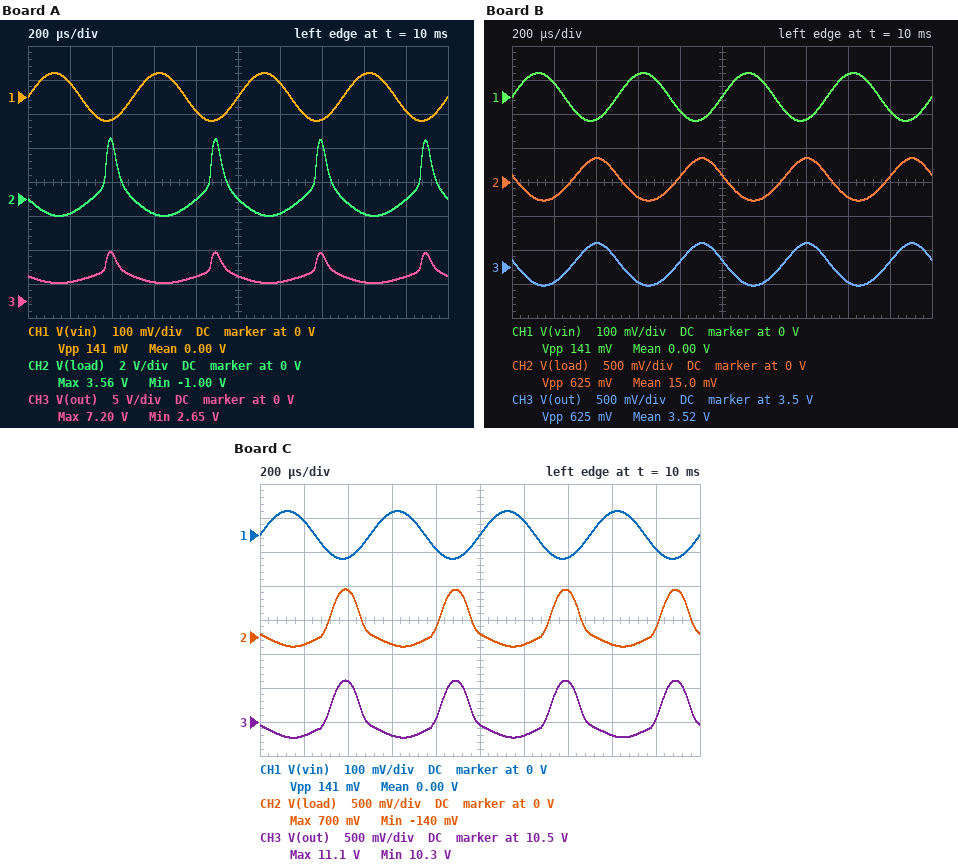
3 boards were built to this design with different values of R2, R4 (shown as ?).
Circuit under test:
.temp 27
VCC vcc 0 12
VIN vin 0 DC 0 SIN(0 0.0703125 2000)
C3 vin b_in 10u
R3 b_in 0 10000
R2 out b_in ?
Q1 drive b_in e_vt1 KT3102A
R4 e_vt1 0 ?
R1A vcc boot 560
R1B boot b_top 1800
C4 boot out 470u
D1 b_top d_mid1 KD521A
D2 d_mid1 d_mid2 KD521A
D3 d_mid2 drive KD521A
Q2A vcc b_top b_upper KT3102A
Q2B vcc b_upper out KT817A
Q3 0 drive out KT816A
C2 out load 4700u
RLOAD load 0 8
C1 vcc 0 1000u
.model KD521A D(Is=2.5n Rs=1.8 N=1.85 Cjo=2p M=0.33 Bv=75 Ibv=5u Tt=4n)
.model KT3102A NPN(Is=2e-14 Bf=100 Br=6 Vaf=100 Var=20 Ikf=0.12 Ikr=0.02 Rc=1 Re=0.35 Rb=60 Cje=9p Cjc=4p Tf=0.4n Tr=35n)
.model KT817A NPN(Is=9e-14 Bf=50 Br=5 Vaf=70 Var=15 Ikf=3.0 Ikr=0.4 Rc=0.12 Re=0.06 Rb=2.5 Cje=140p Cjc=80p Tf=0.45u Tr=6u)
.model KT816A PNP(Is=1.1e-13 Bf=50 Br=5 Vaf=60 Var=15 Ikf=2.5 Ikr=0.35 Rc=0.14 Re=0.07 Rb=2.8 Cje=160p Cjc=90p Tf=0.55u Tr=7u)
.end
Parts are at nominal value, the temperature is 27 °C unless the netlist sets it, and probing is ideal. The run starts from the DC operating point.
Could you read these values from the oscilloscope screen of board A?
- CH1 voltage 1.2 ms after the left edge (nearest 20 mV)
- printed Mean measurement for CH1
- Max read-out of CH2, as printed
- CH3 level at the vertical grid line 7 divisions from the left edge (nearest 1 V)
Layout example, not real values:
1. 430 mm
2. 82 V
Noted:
1. 40 mV
2. 0.00 V
3. 3.56 V
4. 7 V
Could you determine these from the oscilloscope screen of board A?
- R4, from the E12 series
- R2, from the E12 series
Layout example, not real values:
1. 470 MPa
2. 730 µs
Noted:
1. 33 Ω
2. 22 kΩ
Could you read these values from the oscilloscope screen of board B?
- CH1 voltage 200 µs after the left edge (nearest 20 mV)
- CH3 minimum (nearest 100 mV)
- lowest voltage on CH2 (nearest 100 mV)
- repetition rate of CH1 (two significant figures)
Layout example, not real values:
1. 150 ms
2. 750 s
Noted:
1. 40 mV
2. 3.2 V
3. -300 mV
4. 2.0 kHz
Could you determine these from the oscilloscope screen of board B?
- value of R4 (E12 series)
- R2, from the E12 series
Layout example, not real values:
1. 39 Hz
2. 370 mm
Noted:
1. 120 Ω
2. 15 kΩ
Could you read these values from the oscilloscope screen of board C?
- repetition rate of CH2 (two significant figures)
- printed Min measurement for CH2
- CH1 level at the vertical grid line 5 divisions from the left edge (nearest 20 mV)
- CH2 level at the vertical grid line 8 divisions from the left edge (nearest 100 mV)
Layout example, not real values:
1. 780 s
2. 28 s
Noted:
1. 2.0 kHz
2. -140 mV
3. 0 V
4. -100 mV
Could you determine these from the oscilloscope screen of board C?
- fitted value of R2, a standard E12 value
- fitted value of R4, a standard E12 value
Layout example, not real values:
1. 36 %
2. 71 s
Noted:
1. 150 kΩ
2. 120 Ω
